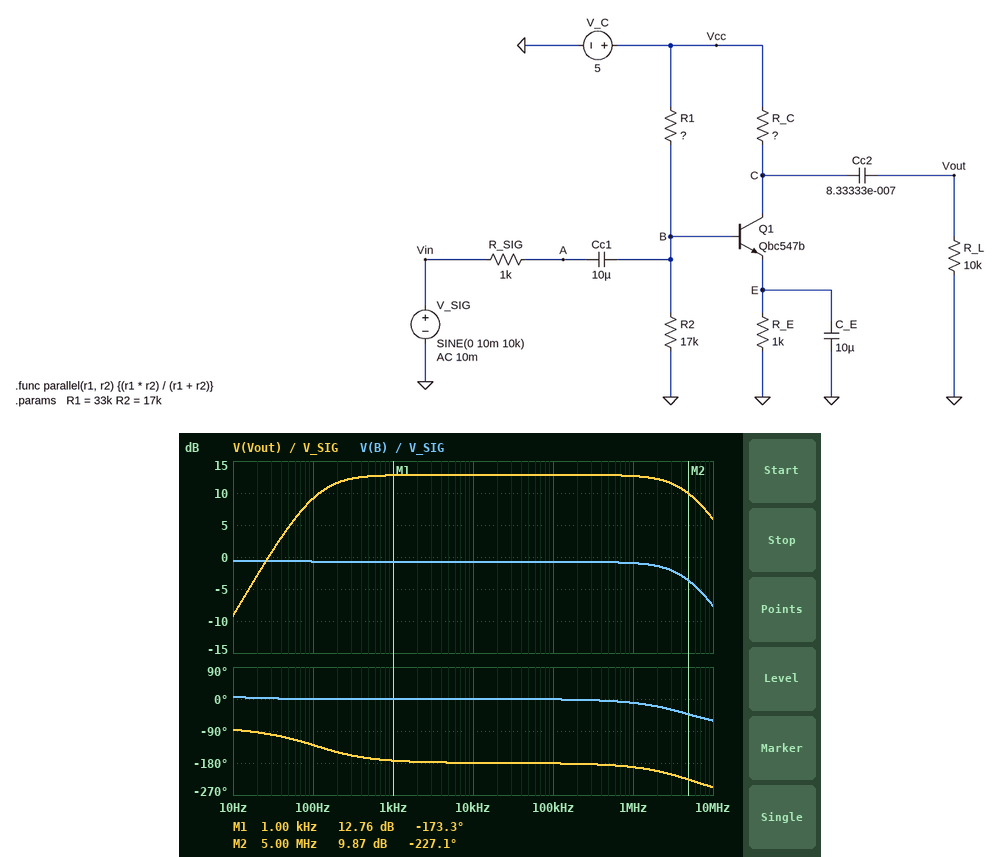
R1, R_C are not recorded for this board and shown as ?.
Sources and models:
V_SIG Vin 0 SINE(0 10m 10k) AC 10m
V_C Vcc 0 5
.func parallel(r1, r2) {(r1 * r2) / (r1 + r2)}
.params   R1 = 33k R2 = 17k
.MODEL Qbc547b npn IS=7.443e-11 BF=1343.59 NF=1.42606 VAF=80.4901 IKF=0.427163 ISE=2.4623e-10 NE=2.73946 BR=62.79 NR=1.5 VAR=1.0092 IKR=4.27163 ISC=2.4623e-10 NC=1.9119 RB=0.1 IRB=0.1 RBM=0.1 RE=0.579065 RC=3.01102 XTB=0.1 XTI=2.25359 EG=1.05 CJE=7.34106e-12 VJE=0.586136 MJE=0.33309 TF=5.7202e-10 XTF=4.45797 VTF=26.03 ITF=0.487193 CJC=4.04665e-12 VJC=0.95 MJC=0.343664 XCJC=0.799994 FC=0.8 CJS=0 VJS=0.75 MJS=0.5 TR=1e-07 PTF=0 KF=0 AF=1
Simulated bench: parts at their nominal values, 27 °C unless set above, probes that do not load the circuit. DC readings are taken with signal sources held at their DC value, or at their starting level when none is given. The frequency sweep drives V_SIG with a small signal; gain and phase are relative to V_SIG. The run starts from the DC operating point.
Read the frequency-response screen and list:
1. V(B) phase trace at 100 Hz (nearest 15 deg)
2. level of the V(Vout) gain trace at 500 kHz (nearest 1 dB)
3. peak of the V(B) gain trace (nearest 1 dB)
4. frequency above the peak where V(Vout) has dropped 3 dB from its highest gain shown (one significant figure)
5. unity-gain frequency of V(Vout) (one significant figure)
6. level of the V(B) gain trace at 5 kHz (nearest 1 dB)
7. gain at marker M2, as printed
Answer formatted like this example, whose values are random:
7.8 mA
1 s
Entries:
0 deg
13 dB
-1 dB
5 MHz
30 Hz
-1 dB
9.87 dB
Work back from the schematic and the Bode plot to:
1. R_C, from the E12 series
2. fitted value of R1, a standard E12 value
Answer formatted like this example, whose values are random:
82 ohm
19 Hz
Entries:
820 Ω
82 kΩ
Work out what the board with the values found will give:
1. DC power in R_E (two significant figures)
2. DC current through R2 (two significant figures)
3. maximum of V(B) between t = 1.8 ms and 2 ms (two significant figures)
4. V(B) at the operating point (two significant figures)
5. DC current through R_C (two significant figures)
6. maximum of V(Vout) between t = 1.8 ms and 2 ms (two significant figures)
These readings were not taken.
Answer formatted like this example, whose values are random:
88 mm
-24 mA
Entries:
66 µW
49 µA
850 mV
840 mV
260 µA
41 mV
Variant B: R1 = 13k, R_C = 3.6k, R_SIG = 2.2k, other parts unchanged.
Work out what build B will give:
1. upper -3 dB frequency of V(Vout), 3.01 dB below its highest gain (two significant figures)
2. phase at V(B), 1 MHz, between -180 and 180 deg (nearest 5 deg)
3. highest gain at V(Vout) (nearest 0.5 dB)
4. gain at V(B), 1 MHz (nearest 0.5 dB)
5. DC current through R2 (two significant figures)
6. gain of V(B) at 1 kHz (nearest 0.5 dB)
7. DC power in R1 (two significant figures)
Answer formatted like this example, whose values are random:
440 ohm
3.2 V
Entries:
130 kHz
-25 deg
-19.0 dB
-37.0 dB
110 µA
-25.5 dB
760 µW
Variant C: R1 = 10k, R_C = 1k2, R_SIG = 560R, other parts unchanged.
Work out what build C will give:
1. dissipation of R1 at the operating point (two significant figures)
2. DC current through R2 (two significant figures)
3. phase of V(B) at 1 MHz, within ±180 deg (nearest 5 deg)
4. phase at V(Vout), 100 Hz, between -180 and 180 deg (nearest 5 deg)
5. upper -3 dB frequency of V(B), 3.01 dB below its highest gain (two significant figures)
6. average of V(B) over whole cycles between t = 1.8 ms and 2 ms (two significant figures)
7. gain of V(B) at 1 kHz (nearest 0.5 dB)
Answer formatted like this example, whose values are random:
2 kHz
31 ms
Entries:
430 µW
170 µA
-35 deg
-120 deg
140 Hz
2.9 V
-16.0 dB
